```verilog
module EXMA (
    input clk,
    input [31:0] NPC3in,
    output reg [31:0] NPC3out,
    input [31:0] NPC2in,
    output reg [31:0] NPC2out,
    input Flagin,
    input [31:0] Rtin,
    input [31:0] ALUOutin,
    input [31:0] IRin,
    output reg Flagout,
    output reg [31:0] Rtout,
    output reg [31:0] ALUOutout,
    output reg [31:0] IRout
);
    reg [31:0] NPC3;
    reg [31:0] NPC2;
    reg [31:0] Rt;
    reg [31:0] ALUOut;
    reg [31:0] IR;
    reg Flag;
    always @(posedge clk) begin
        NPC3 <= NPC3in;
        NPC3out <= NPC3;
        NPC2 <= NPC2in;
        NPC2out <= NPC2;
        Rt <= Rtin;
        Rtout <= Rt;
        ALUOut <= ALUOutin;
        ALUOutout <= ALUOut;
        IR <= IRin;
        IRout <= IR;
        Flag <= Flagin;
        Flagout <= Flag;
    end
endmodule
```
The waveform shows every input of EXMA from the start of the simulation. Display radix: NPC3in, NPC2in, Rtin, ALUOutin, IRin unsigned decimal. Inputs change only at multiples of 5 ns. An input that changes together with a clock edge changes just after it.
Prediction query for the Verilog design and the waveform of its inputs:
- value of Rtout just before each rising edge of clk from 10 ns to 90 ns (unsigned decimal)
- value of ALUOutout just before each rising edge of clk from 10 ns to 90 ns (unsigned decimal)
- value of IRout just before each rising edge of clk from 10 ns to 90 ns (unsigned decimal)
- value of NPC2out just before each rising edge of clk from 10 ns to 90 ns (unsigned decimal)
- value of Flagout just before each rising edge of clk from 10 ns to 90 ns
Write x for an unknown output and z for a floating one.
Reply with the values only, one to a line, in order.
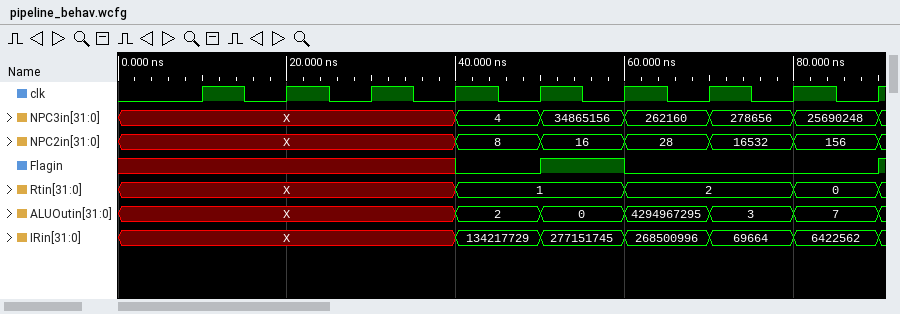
x, x, x, x, x, x, 1, 1, 2
x, x, x, x, x, x, 2, 0, 4294967295
x, x, x, x, x, x, 134217729, 277151745, 268500996
x, x, x, x, x, x, 8, 16, 28
x x x x x x 0 1 0
